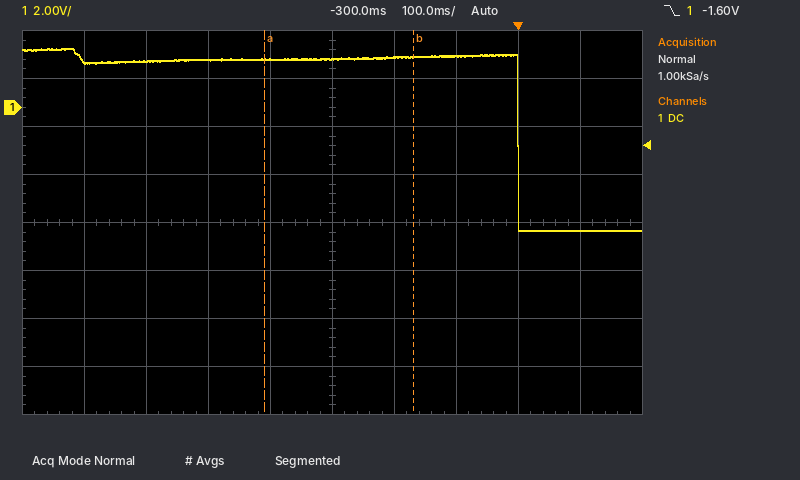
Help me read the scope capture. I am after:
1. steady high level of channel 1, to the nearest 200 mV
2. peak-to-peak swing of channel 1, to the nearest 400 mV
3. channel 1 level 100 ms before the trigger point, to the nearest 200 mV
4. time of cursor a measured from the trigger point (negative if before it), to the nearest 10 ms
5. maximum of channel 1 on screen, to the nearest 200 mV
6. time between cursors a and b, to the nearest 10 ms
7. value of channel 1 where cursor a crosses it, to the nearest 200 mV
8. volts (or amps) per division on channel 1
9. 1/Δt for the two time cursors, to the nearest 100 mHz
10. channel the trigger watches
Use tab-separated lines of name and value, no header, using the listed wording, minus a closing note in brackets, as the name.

steady high level of channel 1, to the nearest 200 mV	2.0 V
peak-to-peak swing of channel 1, to the nearest 400 mV	7.6 V
channel 1 level 100 ms before the trigger point, to the nearest 200 mV	2.2 V
time of cursor a measured from the trigger point (negative if before it), to the nearest 10 ms	-410 ms
maximum of channel 1 on screen, to the nearest 200 mV	2.4 V
time between cursors a and b, to the nearest 10 ms	240 ms
value of channel 1 where cursor a crosses it, to the nearest 200 mV	2.0 V
volts (or amps) per division on channel 1	2 V
1/Δt for the two time cursors, to the nearest 100 mHz	4.2 Hz
channel the trigger watches	channel 1
